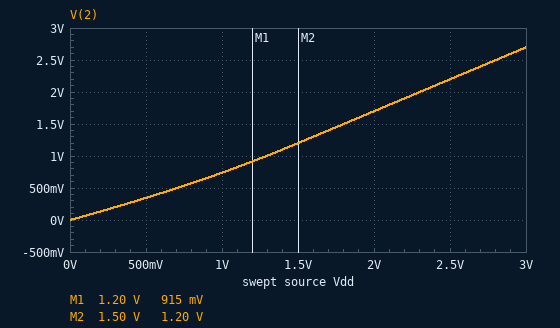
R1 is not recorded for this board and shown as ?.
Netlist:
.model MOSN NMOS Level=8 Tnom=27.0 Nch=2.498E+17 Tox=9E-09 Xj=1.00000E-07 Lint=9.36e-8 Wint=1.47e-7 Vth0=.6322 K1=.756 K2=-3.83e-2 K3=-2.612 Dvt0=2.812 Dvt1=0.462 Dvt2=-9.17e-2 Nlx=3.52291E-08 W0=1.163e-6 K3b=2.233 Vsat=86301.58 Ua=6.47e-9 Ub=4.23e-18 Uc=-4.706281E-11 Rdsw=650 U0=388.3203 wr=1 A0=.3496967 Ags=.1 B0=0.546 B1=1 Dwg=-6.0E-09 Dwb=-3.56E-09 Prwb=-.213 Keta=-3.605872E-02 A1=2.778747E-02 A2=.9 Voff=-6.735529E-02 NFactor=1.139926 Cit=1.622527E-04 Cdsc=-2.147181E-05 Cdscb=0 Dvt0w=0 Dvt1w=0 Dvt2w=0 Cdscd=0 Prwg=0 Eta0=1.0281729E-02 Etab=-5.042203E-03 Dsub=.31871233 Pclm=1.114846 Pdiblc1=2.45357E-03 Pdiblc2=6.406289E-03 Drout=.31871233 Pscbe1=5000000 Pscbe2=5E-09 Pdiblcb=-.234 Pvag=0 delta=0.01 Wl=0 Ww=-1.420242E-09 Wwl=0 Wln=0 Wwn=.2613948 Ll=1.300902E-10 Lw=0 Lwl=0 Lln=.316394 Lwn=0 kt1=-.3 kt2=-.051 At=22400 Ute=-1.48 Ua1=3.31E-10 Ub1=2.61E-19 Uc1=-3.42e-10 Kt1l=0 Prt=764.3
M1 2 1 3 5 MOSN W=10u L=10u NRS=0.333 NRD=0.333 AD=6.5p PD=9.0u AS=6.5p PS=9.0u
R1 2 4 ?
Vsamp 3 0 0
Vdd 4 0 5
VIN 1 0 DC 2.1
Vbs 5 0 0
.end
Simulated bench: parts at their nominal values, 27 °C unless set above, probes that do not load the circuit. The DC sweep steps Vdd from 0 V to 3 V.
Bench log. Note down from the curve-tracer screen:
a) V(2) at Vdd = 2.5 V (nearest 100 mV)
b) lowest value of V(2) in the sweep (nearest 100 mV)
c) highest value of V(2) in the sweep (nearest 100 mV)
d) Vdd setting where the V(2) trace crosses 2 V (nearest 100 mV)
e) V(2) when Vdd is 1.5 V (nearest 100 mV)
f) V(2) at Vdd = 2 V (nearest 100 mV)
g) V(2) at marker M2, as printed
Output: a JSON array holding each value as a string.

["2.2 V", "0 V", "2.7 V", "2.3 V", "1.2 V", "1.7 V", "1.20 V"]
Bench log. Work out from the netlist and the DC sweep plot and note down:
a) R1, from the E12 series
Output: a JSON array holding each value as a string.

["8.2 kΩ"]
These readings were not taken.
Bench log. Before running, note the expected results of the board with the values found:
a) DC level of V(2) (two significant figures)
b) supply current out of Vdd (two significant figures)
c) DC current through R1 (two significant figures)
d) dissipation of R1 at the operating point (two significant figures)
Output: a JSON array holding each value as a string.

["4.7 V", "37 µA", "37 µA", "11 µW"]
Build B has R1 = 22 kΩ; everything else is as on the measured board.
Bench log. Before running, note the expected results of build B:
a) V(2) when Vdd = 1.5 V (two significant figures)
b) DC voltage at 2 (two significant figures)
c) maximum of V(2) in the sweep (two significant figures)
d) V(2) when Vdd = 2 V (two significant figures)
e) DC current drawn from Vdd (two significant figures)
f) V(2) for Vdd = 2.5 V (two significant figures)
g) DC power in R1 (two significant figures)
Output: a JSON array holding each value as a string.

["780 mV", "4.2 V", "2.2 V", "1.2 V", "37 µA", "1.7 V", "30 µW"]
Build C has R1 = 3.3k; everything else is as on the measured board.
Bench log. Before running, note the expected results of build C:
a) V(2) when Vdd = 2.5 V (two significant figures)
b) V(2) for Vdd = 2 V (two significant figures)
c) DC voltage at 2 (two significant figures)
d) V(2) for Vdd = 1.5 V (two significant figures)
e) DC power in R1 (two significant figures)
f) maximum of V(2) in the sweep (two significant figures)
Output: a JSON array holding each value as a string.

["2.4 V", "1.9 V", "4.9 V", "1.4 V", "4.6 µW", "2.9 V"]
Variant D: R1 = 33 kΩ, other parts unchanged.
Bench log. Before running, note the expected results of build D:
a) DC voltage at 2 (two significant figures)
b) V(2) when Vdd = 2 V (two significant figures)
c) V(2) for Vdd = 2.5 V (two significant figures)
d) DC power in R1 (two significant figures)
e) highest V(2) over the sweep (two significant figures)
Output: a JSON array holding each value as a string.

["3.8 V", "870 mV", "1.3 V", "45 µW", "1.8 V"]
